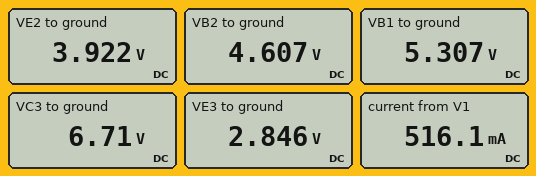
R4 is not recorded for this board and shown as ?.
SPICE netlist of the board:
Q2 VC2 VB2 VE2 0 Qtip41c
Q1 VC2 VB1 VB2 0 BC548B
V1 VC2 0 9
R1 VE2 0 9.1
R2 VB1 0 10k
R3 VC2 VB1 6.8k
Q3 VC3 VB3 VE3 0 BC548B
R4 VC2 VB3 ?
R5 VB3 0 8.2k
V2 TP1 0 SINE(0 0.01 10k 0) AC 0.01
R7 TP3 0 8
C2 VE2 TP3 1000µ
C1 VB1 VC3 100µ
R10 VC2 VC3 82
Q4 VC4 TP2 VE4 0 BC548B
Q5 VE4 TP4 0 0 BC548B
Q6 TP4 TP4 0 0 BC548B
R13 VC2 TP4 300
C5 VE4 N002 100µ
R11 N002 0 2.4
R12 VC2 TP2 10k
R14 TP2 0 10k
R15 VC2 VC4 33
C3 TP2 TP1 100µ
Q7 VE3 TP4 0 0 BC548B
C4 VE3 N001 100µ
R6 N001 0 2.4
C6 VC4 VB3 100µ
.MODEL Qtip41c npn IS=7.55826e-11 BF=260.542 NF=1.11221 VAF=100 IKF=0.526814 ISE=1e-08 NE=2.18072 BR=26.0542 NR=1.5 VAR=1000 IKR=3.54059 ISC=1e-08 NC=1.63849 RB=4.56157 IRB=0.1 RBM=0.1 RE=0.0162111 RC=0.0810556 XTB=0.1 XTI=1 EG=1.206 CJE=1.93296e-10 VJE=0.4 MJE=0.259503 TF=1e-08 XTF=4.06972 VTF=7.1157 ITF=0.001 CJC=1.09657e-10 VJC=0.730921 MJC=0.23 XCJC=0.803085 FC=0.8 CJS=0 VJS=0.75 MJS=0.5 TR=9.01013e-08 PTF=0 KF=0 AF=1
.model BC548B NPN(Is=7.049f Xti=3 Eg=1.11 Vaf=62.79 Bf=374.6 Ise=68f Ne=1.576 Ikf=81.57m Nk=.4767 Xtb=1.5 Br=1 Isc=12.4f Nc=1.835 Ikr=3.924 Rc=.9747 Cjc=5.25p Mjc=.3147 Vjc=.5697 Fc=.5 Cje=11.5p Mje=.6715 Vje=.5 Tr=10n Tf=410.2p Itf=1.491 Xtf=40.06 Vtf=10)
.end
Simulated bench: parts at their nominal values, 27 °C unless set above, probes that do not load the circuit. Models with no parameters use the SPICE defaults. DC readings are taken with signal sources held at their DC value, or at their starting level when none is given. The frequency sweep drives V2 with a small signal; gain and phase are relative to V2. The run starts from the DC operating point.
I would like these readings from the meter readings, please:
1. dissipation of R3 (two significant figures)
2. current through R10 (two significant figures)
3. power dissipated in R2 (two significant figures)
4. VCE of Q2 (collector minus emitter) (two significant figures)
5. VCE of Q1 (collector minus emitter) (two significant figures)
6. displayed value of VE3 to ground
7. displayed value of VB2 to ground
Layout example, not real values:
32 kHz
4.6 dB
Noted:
2.0 mW
28 mA
2.8 mW
5.1 V
4.4 V
2.846 V
4.607 V
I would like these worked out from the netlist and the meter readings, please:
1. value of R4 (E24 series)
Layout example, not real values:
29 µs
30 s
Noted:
10 kΩ
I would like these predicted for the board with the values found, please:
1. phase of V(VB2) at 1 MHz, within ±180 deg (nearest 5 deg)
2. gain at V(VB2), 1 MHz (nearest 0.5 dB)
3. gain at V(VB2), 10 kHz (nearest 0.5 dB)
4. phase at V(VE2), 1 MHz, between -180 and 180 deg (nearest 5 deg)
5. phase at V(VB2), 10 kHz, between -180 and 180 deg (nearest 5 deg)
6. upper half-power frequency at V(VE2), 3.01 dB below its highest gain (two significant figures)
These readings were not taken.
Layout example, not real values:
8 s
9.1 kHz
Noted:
-20 deg
44.5 dB
46.0 dB
-30 deg
5 deg
1.3 MHz
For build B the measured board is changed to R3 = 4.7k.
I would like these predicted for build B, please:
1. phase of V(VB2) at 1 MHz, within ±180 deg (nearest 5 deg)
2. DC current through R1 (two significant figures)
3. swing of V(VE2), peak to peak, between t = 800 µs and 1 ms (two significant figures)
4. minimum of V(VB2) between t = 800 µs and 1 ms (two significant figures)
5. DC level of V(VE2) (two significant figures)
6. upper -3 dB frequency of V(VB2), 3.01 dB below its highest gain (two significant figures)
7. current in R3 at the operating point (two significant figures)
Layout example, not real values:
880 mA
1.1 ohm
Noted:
-15 deg
510 mA
3.5 V
3.4 V
4.7 V
2.3 MHz
620 µA
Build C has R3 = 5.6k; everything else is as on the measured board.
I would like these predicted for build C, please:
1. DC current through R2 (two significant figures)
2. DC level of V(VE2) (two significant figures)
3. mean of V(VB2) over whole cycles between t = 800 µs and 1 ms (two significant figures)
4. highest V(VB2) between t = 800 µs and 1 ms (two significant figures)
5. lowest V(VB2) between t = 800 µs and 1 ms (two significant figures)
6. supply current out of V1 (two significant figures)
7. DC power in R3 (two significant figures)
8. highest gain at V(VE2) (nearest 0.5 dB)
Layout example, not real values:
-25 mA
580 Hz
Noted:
570 µA
4.3 V
5.0 V
6.7 V
3.1 V
560 mA
1.9 mW
45.5 dB
